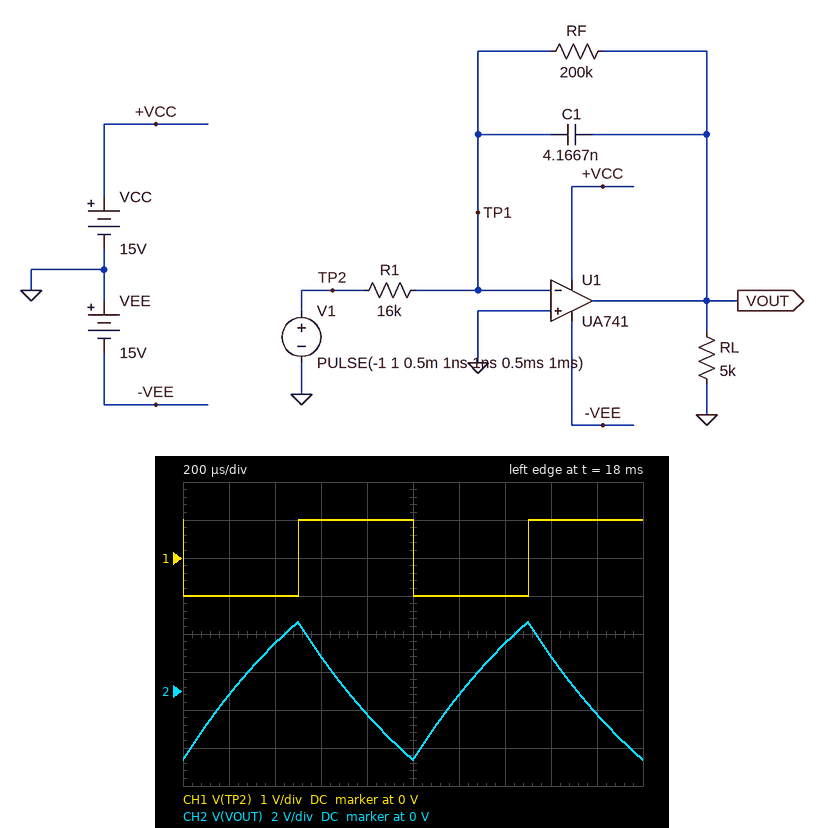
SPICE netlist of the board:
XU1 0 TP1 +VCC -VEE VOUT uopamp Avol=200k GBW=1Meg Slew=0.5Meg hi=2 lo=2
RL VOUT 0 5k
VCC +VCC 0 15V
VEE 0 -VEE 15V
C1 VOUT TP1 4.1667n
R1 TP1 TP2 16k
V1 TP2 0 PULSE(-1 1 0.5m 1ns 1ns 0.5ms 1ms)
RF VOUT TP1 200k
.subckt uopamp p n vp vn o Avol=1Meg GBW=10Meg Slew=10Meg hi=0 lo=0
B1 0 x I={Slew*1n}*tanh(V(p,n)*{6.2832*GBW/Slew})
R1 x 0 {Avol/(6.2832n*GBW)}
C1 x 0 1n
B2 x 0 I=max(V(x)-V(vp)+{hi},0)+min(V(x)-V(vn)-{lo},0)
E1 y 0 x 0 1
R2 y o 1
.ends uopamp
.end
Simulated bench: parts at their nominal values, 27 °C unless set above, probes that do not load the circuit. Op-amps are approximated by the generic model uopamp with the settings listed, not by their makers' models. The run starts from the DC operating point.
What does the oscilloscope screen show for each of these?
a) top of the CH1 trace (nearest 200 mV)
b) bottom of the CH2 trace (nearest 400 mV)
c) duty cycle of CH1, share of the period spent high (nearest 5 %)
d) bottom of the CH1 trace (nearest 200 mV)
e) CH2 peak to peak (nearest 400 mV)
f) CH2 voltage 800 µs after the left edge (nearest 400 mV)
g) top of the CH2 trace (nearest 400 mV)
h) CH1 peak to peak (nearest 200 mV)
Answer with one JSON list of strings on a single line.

["1.0 V", "-3.6 V", "50 %", "-1.0 V", "7.2 V", "-1.2 V", "3.6 V", "2.0 V"]
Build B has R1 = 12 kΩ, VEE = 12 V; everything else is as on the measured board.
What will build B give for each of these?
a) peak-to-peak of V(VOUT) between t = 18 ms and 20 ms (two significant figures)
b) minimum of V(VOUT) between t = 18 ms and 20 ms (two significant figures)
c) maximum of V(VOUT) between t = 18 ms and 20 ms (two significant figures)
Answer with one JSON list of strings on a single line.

["9.7 V", "-4.8 V", "4.8 V"]
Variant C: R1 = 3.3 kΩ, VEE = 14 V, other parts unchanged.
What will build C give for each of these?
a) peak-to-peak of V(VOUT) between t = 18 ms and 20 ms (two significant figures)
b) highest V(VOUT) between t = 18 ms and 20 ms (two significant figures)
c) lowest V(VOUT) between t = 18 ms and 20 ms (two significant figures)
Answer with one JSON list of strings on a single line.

["25 V", "13 V", "-12 V"]
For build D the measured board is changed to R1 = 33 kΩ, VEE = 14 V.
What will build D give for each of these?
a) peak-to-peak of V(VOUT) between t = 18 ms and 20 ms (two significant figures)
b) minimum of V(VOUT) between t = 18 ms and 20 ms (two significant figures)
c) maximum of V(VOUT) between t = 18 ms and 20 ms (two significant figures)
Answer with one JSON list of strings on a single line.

["3.5 V", "-1.8 V", "1.8 V"]
